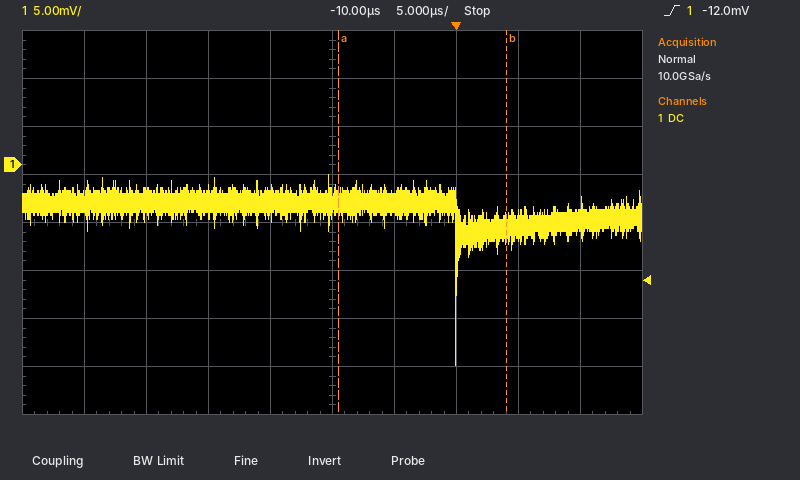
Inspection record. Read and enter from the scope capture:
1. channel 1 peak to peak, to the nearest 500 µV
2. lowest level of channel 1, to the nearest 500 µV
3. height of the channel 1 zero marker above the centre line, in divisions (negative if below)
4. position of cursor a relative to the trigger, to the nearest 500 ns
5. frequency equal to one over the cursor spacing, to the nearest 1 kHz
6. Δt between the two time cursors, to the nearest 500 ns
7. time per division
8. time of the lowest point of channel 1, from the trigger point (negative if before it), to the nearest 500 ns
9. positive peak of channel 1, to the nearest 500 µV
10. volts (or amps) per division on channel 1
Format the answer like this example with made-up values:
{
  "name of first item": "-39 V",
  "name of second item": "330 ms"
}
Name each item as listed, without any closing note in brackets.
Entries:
{
  "channel 1 peak to peak, to the nearest 500 µV": "20.0 mV",
  "lowest level of channel 1, to the nearest 500 µV": "-21.0 mV",
  "height of the channel 1 zero marker above the centre line, in divisions": "+1.2 div",
  "position of cursor a relative to the trigger, to the nearest 500 ns": "-9.5 µs",
  "frequency equal to one over the cursor spacing, to the nearest 1 kHz": "74 kHz",
  "Δt between the two time cursors, to the nearest 500 ns": "13.5 µs",
  "time per division": "5 µs",
  "time of the lowest point of channel 1, from the trigger point (negative if before it), to the nearest 500 ns": "0.0 µs",
  "positive peak of channel 1, to the nearest 500 µV": "-1.0 mV",
  "volts (or amps) per division on channel 1": "5 mV"
}
